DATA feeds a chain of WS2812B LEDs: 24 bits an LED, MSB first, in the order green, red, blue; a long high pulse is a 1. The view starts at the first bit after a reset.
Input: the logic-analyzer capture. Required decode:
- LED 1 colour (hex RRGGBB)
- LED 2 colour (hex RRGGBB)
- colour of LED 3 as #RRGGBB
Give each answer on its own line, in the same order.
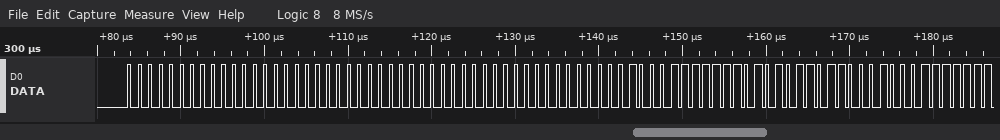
#000000
#000000
#EA8FD8
